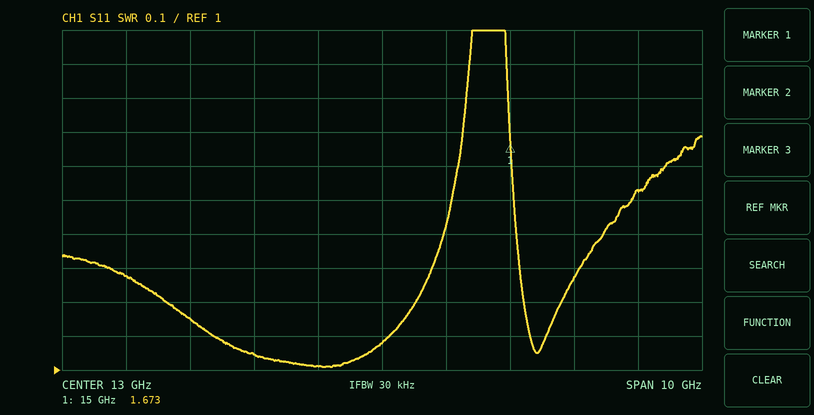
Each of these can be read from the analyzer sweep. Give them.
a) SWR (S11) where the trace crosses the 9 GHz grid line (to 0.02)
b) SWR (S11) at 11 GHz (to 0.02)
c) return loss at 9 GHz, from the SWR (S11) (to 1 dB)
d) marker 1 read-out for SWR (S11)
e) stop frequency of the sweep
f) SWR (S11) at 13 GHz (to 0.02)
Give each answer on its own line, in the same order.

1.28
1.04
18 dB
1.673
18 GHz
1.08
